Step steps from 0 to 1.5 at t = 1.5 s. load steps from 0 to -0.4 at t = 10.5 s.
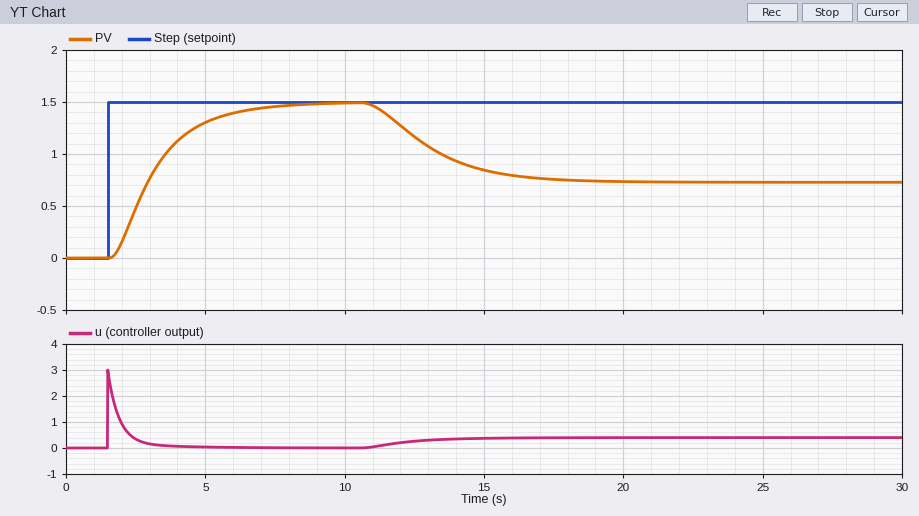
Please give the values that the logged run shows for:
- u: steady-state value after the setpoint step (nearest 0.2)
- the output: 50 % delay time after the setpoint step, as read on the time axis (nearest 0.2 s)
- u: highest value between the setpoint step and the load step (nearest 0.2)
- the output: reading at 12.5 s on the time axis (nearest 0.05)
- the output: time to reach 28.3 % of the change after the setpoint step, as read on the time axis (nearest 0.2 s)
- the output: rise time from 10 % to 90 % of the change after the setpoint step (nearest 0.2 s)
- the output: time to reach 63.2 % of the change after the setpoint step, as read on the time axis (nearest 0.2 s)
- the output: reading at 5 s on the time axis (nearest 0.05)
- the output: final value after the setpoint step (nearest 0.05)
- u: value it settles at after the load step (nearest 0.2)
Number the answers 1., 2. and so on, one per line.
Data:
1. 0.0
2. 3.0 s
3. 3.0
4. 1.15
5. 2.4 s
6. 3.4 s
7. 3.4 s
8. 1.30
9. 1.50
10. 0.4
